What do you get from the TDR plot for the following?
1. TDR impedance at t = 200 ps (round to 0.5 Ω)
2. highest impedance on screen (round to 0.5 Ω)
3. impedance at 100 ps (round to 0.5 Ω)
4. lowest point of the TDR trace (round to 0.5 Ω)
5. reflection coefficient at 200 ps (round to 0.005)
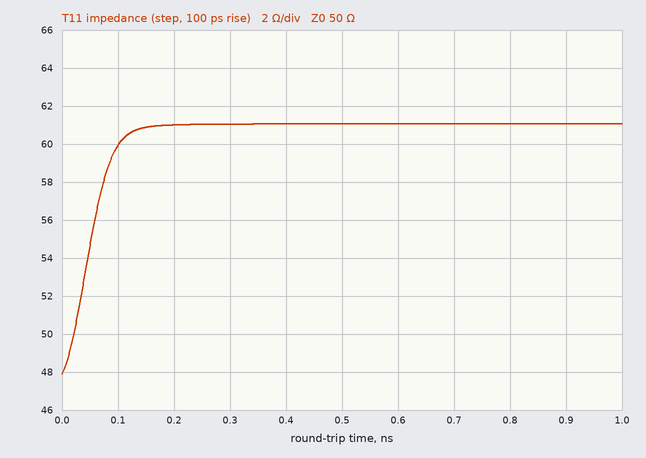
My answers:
61.0 Ω
61.0 Ω
60.0 Ω
48.0 Ω
+0.100
